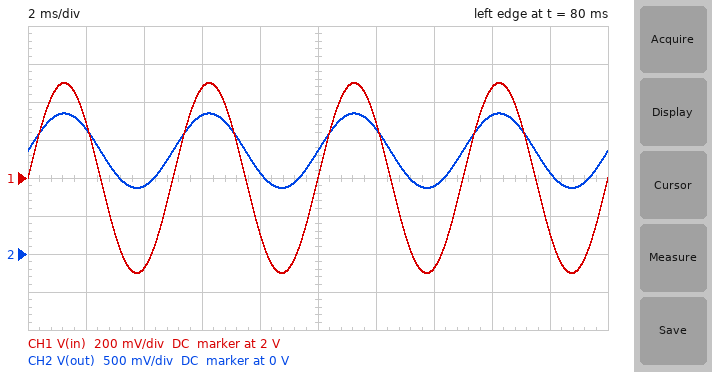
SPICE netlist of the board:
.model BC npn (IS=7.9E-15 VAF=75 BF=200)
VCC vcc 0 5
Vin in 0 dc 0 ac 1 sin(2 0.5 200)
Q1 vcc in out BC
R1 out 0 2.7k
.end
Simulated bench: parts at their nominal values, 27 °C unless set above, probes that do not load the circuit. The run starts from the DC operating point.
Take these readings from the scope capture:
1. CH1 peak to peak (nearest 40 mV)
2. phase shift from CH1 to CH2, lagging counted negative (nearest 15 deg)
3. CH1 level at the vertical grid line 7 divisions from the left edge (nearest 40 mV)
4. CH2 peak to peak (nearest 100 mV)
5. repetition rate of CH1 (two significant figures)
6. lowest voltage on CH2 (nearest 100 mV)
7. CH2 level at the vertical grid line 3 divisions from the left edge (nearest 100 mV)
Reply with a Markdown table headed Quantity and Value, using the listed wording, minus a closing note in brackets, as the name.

| Quantity | Value |
|---|---|
| CH1 peak to peak | 1.00 V |
| phase shift from CH1 to CH2, lagging counted negative | 0 deg |
| CH1 level at the vertical grid line 7 divisions from the left edge | 1.52 V |
| CH2 peak to peak | 1.0 V |
| repetition rate of CH1 | 200 Hz |
| lowest voltage on CH2 | 900 mV |
| CH2 level at the vertical grid line 3 divisions from the left edge | 1.8 V |
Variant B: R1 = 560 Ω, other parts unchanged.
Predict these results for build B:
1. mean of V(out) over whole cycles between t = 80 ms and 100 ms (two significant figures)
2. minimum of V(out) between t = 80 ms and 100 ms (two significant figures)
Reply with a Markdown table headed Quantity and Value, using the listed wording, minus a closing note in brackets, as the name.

| Quantity | Value |
|---|---|
| mean of V(out) over whole cycles between t = 80 ms and 100 ms | 1.3 V |
| minimum of V(out) between t = 80 ms and 100 ms | 830 mV |
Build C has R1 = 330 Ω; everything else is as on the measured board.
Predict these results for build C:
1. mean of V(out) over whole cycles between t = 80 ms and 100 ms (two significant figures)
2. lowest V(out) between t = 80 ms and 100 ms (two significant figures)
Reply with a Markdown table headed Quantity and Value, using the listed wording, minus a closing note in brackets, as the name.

| Quantity | Value |
|---|---|
| mean of V(out) over whole cycles between t = 80 ms and 100 ms | 1.3 V |
| lowest V(out) between t = 80 ms and 100 ms | 820 mV |
